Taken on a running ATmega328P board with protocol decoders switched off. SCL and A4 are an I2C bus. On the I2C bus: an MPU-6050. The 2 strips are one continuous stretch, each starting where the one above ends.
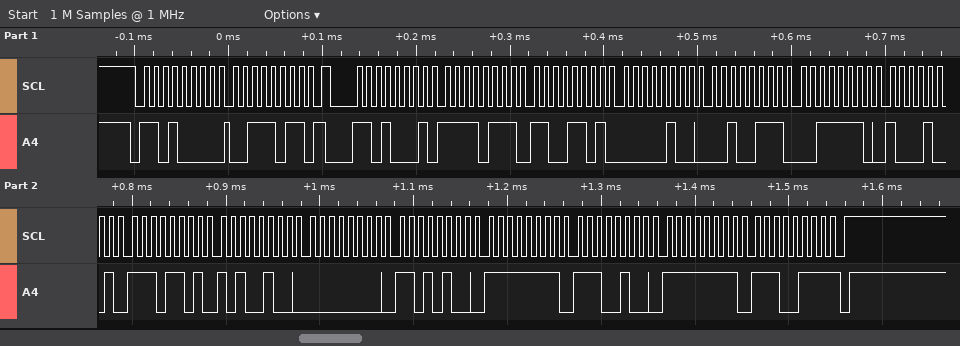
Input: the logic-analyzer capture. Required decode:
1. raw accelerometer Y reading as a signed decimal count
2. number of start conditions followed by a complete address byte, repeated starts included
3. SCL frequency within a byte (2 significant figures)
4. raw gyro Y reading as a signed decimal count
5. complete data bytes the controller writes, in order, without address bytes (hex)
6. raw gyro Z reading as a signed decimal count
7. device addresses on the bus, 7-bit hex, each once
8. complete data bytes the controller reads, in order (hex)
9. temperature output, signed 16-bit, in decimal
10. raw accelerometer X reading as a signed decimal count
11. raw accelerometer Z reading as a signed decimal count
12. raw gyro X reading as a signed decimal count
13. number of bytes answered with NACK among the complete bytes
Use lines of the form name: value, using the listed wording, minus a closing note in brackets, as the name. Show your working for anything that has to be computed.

raw accelerometer Y reading as a signed decimal count: 0x0427 = 1063
number of start conditions followed by a complete address byte, repeated starts included: 2
SCL frequency within a byte: 100 kHz
raw gyro Y reading as a signed decimal count: 0xFFE4 = -28
complete data bytes the controller writes, in order, without address bytes: 3B
raw gyro Z reading as a signed decimal count: 0xFFE7 = -25
device addresses on the bus, 7-bit hex, each once: 0x68
complete data bytes the controller reads, in order: F7 CD 04 27 3E 89 ED A4 00 D4 FF E4 FF E7
temperature output, signed 16-bit, in decimal: 0xEDA4 = -4700
raw accelerometer X reading as a signed decimal count: 0xF7CD = -2099
raw accelerometer Z reading as a signed decimal count: 0x3E89 = 16009
raw gyro X reading as a signed decimal count: 0x00D4 = 212
number of bytes answered with NACK among the complete bytes: 1
